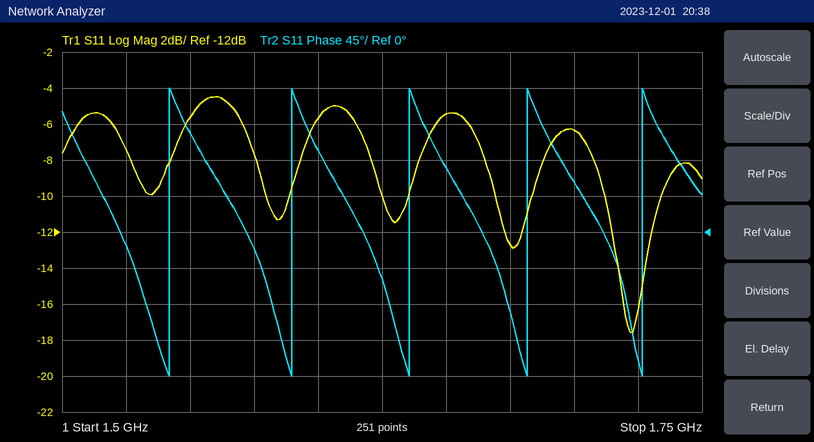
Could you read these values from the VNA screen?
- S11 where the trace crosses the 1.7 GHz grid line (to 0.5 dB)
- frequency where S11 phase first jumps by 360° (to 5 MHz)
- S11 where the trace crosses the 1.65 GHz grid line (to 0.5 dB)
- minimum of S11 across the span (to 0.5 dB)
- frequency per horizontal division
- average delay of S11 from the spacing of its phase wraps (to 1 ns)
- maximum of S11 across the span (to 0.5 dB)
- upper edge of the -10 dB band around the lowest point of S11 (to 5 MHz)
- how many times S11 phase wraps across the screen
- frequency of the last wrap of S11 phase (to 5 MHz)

-6.5 dB
1.540 GHz
-5.5 dB
-17.5 dB
25 MHz
22 ns
-4.5 dB
1.735 GHz
5
1.725 GHz
